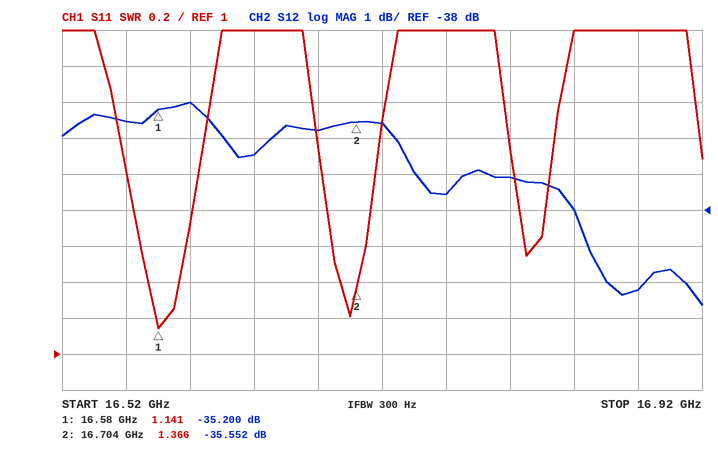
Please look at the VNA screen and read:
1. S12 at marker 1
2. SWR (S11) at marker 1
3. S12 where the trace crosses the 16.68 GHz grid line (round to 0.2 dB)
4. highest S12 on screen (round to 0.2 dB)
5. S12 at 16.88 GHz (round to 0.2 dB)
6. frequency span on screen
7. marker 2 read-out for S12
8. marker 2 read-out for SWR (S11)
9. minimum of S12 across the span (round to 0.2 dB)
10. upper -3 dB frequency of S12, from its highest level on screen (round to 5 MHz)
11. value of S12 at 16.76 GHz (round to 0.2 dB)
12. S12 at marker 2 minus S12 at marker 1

-35.200 dB
1.141
-35.8 dB
-35.0 dB
-40.2 dB
400 MHz
-35.552 dB
1.366
-40.6 dB
16.840 GHz
-37.6 dB
-0.352 dB
